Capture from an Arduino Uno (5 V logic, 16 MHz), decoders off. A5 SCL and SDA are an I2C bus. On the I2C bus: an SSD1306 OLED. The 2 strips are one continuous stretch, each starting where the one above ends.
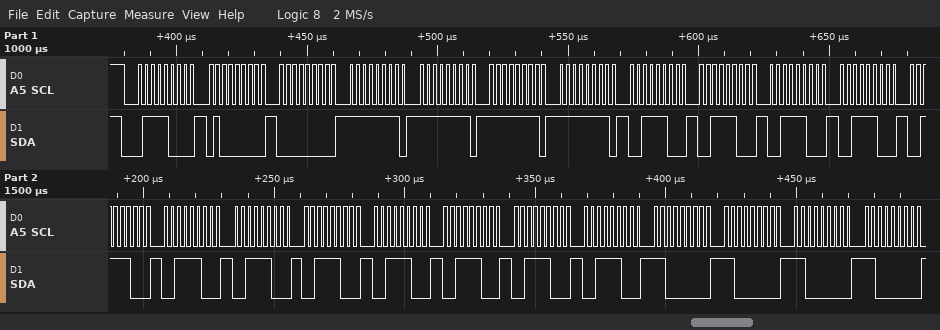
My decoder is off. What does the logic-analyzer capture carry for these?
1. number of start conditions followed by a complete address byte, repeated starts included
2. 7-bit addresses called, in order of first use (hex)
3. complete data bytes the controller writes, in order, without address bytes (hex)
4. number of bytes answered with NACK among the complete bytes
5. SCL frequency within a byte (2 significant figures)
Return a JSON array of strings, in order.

["1", "0x3C", "40 00 FF FF FF FF 3C 3C 3C 3C 3C 3C 3C 3C 3C 3C 3C 3C C0 C0 C0 C0", "0", "400 kHz"]
